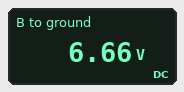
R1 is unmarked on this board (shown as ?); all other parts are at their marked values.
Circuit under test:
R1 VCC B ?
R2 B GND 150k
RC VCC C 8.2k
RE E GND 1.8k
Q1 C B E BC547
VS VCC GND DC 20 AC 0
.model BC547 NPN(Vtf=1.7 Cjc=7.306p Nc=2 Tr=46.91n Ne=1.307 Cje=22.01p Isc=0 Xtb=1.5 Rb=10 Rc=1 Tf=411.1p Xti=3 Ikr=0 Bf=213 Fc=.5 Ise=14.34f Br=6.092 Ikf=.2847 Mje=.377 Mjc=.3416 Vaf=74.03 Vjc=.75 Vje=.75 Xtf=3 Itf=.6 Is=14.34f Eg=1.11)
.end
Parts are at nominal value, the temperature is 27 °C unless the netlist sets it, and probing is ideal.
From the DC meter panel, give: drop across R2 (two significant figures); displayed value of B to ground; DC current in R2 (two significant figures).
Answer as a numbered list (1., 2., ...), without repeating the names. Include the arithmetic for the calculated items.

1. 6.66 V = 6.7 V
2. 6.66 V
3. (6.66 V) / 150 kΩ = 44 µA
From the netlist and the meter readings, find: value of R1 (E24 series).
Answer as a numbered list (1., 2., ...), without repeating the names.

1. 8.2 kΩ
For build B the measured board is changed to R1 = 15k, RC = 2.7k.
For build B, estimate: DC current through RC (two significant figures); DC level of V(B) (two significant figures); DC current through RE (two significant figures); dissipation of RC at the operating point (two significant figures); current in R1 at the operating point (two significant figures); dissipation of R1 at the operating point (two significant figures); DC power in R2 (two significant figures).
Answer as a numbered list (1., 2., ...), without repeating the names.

1. 4.2 mA
2. 9.4 V
3. 4.8 mA
4. 47 mW
5. 710 µA
6. 7.5 mW
7. 590 µW
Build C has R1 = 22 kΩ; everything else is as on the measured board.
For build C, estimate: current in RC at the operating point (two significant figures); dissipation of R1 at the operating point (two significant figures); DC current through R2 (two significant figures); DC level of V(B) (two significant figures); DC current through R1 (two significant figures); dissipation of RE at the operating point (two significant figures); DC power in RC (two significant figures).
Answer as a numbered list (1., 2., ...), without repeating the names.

1. 1.9 mA
2. 9.9 mW
3. 35 µA
4. 5.2 V
5. 670 µA
6. 11 mW
7. 29 mW
